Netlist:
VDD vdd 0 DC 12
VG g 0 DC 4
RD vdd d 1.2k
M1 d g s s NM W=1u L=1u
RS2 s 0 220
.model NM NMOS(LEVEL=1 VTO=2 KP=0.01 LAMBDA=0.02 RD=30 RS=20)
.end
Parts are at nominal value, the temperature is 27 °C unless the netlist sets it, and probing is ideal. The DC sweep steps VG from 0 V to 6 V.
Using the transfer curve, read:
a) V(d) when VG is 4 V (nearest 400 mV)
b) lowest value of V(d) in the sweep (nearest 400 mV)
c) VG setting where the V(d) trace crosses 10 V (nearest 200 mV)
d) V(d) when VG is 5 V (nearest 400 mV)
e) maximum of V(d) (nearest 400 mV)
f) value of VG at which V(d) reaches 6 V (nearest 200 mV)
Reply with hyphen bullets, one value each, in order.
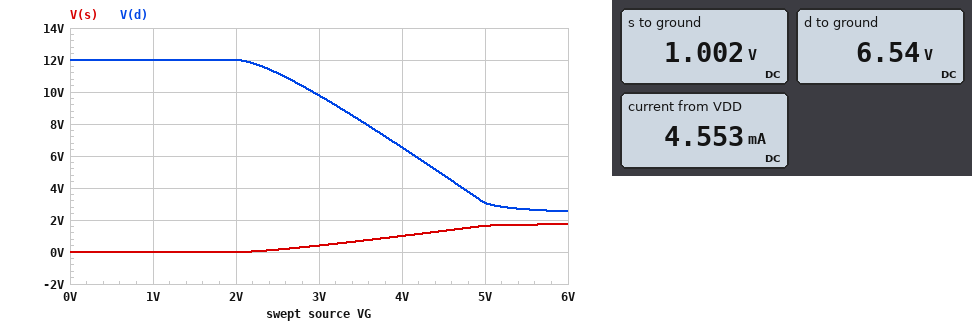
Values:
- 6.4 V
- 2.4 V
- 3.0 V
- 3.2 V
- 12.0 V
- 4.2 V
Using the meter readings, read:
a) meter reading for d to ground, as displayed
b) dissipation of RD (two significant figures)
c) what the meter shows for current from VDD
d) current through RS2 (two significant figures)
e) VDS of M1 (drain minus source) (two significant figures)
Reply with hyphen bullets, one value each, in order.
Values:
- 6.54 V
- 25 mW
- 4.553 mA
- 4.6 mA
- 5.5 V
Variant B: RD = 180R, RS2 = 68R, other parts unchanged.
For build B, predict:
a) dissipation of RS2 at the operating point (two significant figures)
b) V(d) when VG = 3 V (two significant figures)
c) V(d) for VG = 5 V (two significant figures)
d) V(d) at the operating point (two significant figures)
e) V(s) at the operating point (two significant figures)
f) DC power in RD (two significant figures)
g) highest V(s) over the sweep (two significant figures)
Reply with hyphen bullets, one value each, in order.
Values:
- 5.3 mW
- 11 V
- 9.2 V
- 10 V
- 600 mV
- 14 mW
- 1.5 V
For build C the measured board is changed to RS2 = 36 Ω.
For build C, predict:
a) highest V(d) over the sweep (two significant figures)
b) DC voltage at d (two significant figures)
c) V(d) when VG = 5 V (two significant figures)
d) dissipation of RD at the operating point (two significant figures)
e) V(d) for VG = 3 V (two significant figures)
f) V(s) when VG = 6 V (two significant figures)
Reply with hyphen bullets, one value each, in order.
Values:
- 12 V
- 1.5 V
- 1.2 V
- 92 mW
- 7.6 V
- 330 mV
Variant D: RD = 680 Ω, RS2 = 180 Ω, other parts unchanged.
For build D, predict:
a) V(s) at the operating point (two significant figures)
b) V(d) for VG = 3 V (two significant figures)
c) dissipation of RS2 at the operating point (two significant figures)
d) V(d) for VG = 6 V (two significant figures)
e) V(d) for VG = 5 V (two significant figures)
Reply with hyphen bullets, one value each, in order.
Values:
- 940 mV
- 11 V
- 4.9 mW
- 3.9 V
- 6.1 V
